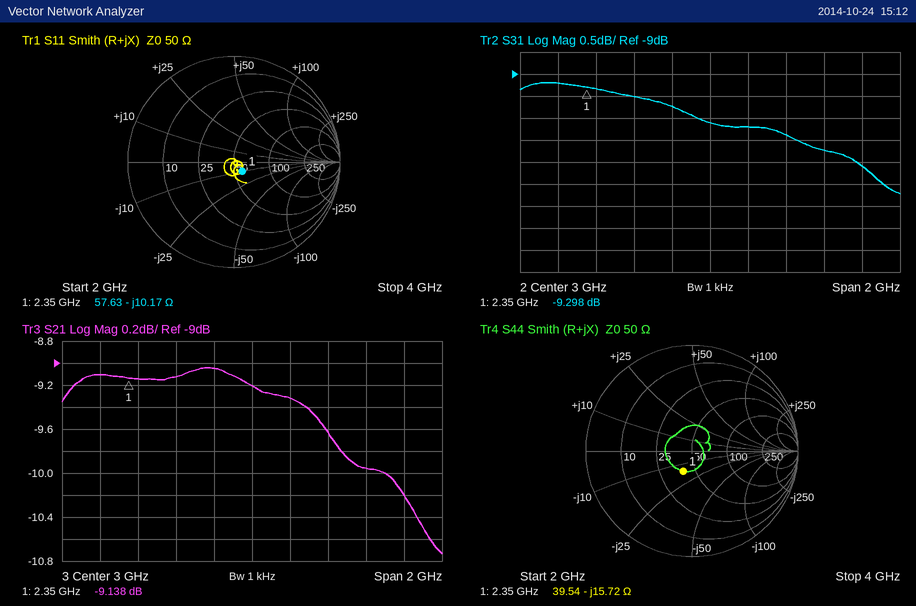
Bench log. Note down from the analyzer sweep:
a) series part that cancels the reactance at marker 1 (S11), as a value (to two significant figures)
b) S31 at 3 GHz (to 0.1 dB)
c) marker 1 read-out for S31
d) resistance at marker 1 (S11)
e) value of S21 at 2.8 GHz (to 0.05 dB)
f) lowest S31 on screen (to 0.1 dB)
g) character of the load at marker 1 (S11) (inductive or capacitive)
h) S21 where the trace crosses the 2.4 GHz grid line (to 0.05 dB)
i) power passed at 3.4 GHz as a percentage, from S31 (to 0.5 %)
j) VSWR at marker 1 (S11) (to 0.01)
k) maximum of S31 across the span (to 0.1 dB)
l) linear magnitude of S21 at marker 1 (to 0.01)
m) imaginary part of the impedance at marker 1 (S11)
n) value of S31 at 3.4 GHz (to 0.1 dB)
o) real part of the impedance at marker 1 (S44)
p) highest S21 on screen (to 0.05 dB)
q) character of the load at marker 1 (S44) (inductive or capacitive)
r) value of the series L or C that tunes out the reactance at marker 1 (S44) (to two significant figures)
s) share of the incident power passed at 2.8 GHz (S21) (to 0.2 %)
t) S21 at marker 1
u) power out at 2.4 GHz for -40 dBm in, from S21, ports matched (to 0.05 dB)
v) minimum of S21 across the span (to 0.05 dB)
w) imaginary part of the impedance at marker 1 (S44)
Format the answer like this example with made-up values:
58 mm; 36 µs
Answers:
690 pH; -10.1 dB; -9.298 dB; 57.63 Ω; -9.05 dB; -11.7 dB; capacitive; -9.15 dB; 9.0 %; 1.27; -9.2 dB; 0.35; -10.17 Ω; -10.4 dB; 39.54 Ω; -9.05 dB; capacitive; 1.1 nH; 12.4 %; -9.138 dB; -49.15 dBm; -10.75 dB; -15.72 Ω
